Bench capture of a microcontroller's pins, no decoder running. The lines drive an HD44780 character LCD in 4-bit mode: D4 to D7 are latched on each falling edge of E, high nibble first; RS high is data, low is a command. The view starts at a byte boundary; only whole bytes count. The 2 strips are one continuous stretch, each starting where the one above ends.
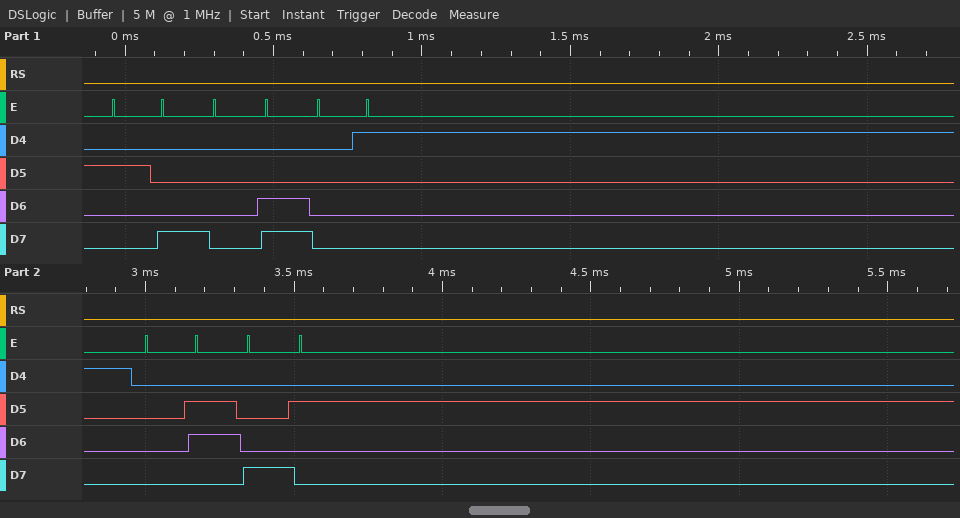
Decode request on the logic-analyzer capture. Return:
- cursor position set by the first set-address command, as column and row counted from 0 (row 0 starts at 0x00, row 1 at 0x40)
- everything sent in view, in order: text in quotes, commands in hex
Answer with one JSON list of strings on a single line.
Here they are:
["column 2, row 0", "0x28 0x0C 0x01 0x06 0x82"]
